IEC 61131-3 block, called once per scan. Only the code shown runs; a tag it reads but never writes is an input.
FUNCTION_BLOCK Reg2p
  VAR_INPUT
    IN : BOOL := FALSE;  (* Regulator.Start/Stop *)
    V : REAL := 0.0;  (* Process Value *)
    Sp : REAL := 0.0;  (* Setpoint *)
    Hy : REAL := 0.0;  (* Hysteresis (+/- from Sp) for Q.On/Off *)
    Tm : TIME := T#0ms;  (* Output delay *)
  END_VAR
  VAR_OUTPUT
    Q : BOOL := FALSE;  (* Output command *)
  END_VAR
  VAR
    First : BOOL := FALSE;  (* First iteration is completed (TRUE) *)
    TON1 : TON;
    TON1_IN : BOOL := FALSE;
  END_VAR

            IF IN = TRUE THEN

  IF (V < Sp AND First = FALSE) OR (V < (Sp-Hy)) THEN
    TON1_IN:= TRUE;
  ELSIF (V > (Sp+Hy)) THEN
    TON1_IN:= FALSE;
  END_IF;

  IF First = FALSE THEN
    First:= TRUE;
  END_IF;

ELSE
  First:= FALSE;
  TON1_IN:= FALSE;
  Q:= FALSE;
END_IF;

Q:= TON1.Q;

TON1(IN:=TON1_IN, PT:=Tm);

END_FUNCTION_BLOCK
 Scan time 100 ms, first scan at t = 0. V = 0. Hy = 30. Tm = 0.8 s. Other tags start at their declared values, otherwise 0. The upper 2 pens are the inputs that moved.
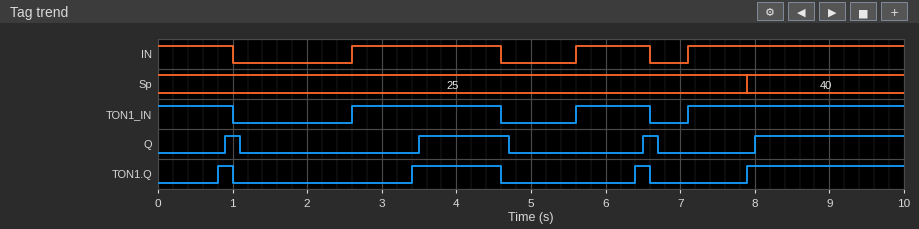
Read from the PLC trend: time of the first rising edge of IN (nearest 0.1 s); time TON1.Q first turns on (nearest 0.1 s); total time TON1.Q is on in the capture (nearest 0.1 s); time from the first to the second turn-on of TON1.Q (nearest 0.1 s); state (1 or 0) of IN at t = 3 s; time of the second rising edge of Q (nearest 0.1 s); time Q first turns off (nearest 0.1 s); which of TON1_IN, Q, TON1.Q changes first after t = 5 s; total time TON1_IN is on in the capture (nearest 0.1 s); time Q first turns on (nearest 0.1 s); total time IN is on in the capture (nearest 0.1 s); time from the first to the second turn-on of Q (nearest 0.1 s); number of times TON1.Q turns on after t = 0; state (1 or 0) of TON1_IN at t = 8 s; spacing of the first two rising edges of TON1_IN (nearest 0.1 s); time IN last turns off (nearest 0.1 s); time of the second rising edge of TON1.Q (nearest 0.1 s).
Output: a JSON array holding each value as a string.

["2.6 s", "0.8 s", "3.7 s", "2.6 s", "1", "3.5 s", "1.1 s", "TON1_IN", "6.9 s", "0.9 s", "6.9 s", "2.6 s", "4", "1", "3.0 s", "6.6 s", "3.4 s"]
